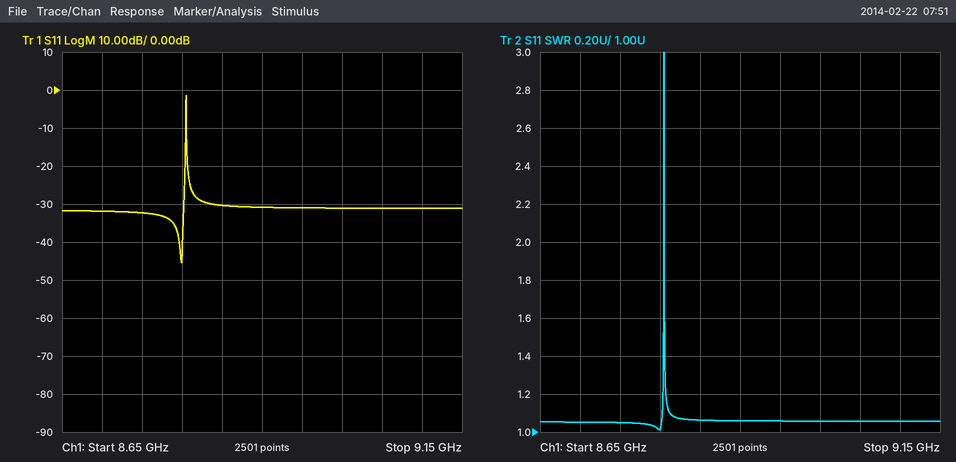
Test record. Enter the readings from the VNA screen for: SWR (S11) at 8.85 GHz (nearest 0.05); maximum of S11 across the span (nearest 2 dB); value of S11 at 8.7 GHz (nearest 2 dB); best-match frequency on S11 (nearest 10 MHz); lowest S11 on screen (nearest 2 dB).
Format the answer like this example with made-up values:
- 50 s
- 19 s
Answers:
- 1.05
- -2 dB
- -32 dB
- 8.80 GHz
- -46 dB
